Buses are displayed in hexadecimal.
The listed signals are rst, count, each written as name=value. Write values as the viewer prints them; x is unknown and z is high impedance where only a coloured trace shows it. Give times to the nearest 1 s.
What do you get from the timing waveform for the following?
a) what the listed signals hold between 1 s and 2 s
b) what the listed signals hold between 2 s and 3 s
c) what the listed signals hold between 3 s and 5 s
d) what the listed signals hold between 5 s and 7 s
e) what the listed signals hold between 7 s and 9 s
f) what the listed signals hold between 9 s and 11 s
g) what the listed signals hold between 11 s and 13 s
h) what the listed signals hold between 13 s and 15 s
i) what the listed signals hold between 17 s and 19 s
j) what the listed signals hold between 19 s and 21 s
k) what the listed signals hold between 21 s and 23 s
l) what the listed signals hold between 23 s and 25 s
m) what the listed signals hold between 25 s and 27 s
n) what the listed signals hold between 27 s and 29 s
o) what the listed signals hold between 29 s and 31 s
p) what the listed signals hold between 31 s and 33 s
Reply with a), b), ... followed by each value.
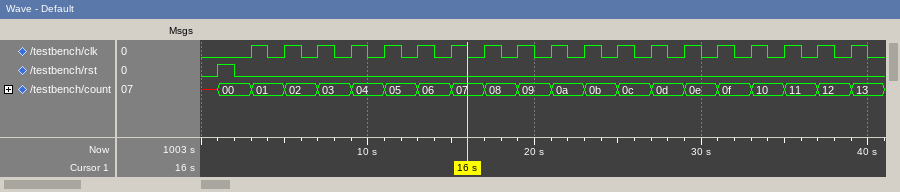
a) rst=1, count=00
b) rst=0, count=00
c) rst=0, count=01
d) rst=0, count=02
e) rst=0, count=03
f) rst=0, count=04
g) rst=0, count=05
h) rst=0, count=06
i) rst=0, count=08
j) rst=0, count=09
k) rst=0, count=0a
l) rst=0, count=0b
m) rst=0, count=0c
n) rst=0, count=0d
o) rst=0, count=0e
p) rst=0, count=0f
